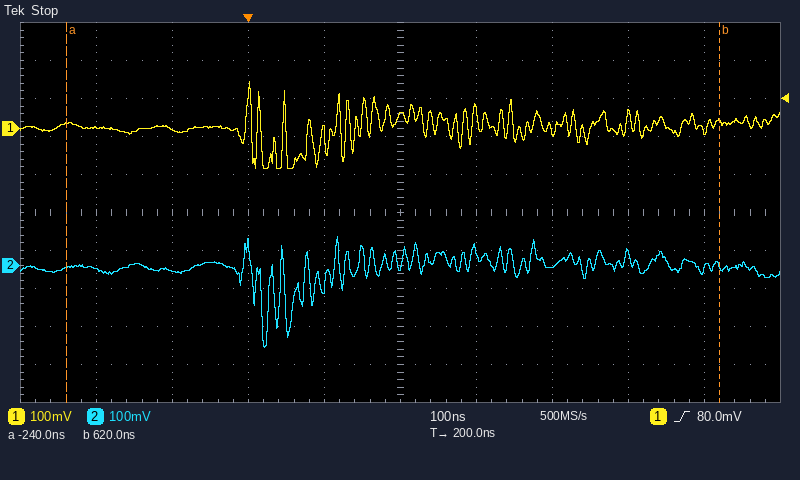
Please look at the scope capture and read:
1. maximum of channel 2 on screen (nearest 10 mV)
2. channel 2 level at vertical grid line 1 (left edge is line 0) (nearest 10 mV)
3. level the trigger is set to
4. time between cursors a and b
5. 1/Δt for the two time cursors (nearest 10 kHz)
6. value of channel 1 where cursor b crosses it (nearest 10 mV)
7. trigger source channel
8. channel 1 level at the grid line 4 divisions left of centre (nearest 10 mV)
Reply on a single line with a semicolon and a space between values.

80 mV; -10 mV; 80.0 mV; 860 ns; 1.16 MHz; 20 mV; channel 1; 0 mV
